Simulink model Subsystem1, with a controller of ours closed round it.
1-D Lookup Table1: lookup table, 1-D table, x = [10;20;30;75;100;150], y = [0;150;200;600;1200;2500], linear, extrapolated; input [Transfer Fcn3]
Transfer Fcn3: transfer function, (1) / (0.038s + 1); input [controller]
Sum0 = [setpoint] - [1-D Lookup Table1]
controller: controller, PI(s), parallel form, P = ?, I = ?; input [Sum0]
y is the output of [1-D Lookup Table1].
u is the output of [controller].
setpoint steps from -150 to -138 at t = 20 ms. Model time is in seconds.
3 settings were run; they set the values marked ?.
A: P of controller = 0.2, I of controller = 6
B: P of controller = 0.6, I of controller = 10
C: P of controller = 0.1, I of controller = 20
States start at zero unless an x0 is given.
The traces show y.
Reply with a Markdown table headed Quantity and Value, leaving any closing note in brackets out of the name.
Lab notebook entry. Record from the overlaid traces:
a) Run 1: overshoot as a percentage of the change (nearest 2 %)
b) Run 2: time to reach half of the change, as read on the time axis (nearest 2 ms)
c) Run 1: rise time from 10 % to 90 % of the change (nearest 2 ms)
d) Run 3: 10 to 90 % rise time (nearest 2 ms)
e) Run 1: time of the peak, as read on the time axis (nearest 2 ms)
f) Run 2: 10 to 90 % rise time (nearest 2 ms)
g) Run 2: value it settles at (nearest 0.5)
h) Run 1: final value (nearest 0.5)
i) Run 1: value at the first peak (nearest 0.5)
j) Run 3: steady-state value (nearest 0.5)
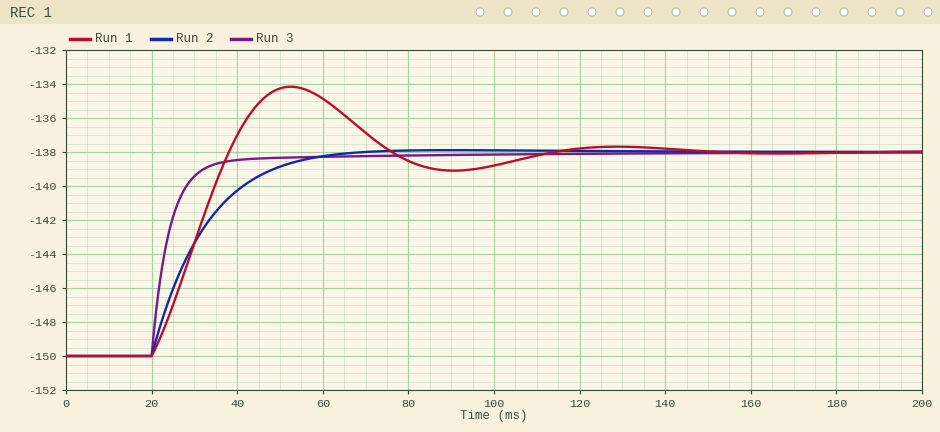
| Quantity | Value |
|---|---|
| Run 1: overshoot as a percentage of the change | 32 % |
| Run 2: time to reach half of the change, as read on the time axis | 28 ms |
| Run 1: rise time from 10 % to 90 % of the change | 14 ms |
| Run 3: 10 to 90 % rise time | 10 ms |
| Run 1: time of the peak, as read on the time axis | 52 ms |
| Run 2: 10 to 90 % rise time | 26 ms |
| Run 2: value it settles at | -138.0 |
| Run 1: final value | -138.0 |
| Run 1: value at the first peak | -134.0 |
| Run 3: steady-state value | -138.0 |
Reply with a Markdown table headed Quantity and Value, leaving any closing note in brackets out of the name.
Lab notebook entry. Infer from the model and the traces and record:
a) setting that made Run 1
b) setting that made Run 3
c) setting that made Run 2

| Quantity | Value |
|---|---|
| setting that made Run 1 | C |
| setting that made Run 3 | B |
| setting that made Run 2 | A |
